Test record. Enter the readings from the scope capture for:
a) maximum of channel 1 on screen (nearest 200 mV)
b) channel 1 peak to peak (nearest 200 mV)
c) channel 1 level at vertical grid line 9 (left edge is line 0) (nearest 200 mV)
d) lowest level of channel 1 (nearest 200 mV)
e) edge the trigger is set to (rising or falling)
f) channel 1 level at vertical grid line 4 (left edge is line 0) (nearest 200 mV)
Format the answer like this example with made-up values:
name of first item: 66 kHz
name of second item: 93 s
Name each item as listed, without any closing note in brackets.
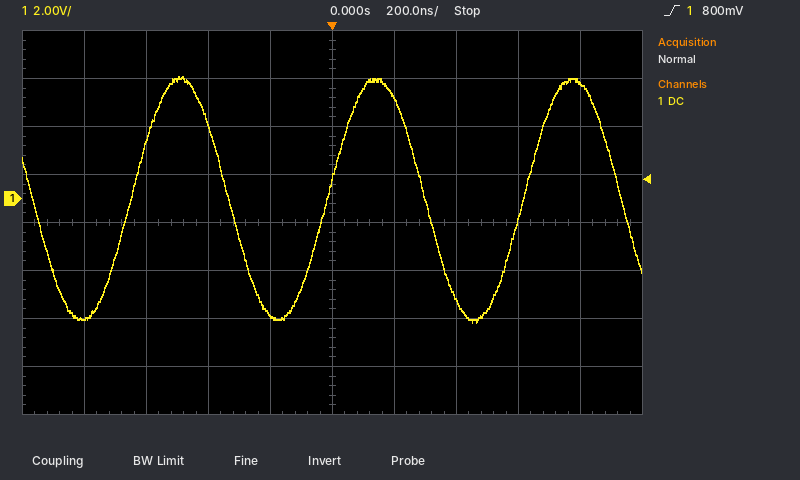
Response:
maximum of channel 1 on screen: 5.0 V
channel 1 peak to peak: 10.2 V
channel 1 level at vertical grid line 9 (left edge is line 0): 4.8 V
lowest level of channel 1: -5.2 V
edge the trigger is set to: rising
channel 1 level at vertical grid line 4 (left edge is line 0): -4.8 V
